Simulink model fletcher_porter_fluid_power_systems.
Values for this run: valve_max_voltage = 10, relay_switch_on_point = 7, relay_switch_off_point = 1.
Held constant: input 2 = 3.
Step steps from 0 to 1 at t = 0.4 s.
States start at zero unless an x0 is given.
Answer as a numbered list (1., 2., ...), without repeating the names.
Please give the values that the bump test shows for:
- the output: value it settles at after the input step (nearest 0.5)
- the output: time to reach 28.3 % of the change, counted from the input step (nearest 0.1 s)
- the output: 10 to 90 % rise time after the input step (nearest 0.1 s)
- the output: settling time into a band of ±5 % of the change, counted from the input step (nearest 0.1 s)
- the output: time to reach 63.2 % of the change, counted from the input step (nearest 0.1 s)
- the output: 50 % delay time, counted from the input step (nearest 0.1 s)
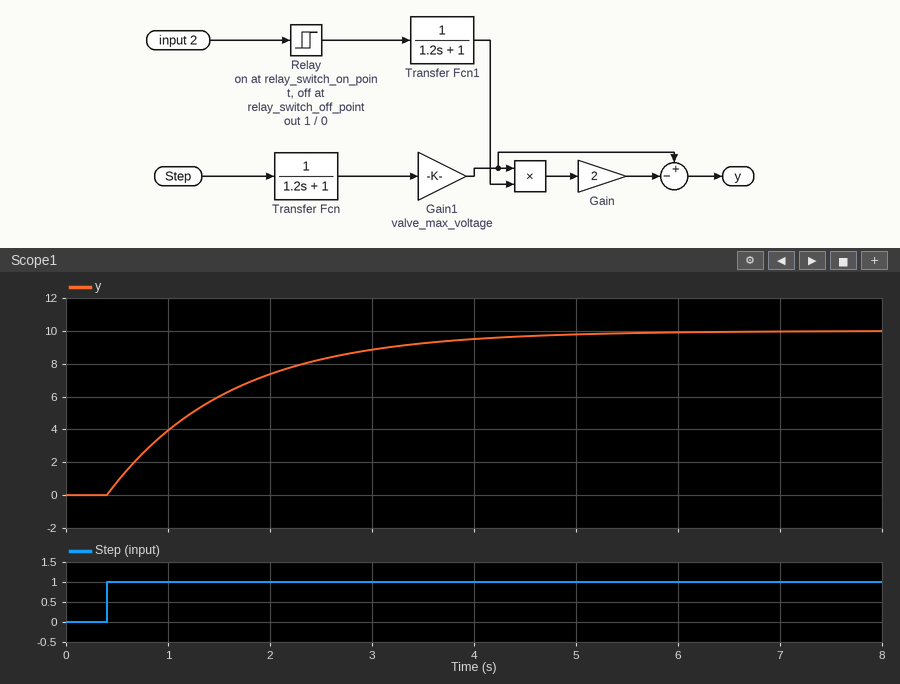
1. 10.0
2. 0.4 s
3. 2.6 s
4. 3.6 s
5. 1.2 s
6. 0.8 s
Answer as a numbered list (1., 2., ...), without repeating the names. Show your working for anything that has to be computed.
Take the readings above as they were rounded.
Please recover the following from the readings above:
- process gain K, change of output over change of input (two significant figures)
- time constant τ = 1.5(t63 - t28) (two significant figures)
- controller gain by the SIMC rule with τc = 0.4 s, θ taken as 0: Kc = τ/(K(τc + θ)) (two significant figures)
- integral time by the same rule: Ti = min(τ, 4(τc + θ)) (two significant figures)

1. (10 - 0) / 1 = 10
2. 1.5 × (1.2 - 0.4) = 1.2 s
3. 1.2 / (10 × (0.4 + 0)) = 0.30
4. min(1.2, 4 × (0.4 + 0)) = 1.2 s
